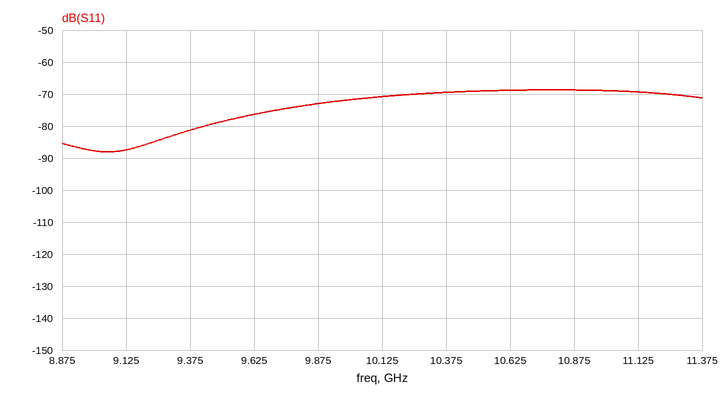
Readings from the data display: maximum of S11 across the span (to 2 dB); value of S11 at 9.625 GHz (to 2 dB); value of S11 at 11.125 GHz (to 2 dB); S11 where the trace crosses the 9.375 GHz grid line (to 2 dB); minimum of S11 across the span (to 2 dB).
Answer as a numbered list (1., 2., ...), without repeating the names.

1. -68 dB
2. -76 dB
3. -70 dB
4. -82 dB
5. -88 dB
